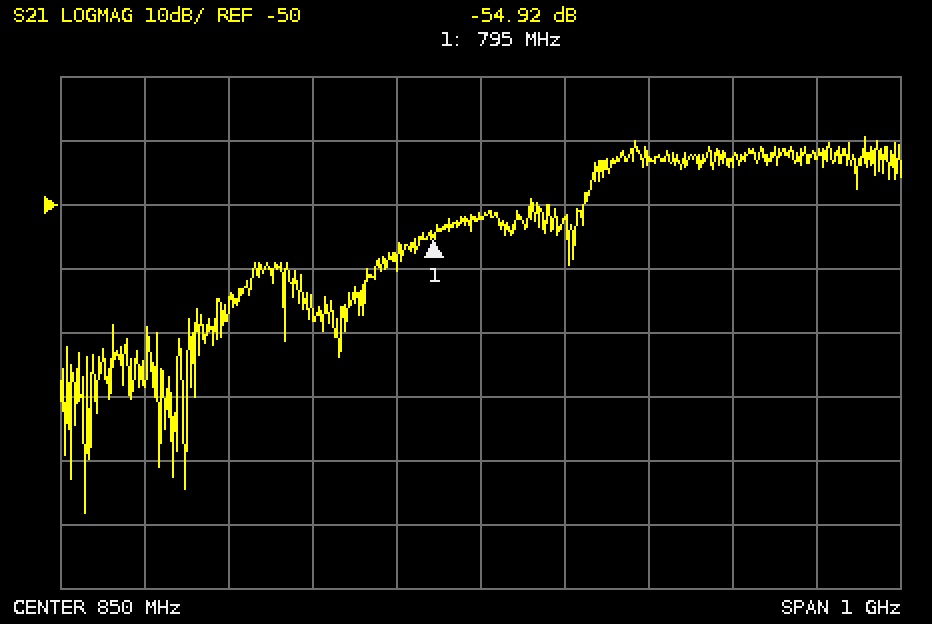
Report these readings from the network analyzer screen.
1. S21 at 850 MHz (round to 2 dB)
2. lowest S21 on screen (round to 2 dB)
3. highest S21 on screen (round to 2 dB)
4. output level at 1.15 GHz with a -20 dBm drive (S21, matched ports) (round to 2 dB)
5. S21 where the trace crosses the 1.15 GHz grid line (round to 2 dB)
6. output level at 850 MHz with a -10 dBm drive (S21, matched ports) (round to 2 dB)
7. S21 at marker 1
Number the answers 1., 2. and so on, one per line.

1. -52 dB
2. -98 dB
3. -40 dB
4. -64 dBm
5. -44 dB
6. -62 dBm
7. -54.92 dB
